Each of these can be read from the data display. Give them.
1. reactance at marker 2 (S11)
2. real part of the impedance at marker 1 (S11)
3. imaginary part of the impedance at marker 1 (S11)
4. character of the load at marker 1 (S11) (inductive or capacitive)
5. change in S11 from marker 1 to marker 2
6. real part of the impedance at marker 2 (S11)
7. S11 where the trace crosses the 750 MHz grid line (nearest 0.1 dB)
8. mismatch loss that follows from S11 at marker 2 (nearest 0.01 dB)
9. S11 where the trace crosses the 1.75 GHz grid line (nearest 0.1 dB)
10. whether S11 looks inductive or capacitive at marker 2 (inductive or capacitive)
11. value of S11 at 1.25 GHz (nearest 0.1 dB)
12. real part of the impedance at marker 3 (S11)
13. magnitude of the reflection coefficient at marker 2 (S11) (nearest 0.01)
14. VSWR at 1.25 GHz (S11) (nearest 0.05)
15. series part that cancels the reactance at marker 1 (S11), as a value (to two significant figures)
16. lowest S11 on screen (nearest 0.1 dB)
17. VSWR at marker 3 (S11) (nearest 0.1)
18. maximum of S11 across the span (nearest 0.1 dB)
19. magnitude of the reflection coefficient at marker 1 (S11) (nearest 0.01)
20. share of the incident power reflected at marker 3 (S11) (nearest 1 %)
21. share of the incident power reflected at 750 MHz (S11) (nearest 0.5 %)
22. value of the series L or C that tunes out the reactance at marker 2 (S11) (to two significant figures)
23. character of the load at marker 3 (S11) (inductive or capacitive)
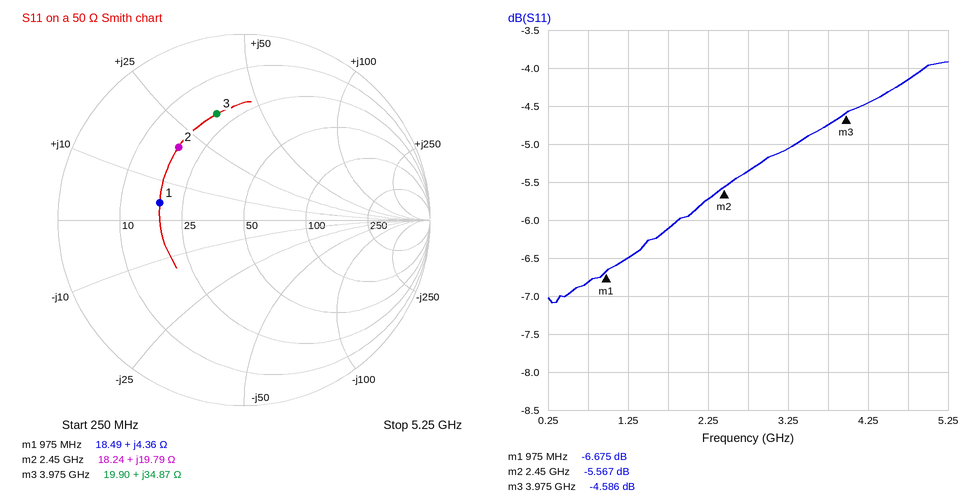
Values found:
+19.79 Ω
18.49 Ω
+4.36 Ω
inductive
1.108 dB
18.24 Ω
-6.8 dB
1.41 dB
-6.1 dB
inductive
-6.5 dB
19.90 Ω
0.53
2.80
37 pF
-7.1 dB
3.9
-3.9 dB
0.46
35 %
21.0 %
3.3 pF
inductive
